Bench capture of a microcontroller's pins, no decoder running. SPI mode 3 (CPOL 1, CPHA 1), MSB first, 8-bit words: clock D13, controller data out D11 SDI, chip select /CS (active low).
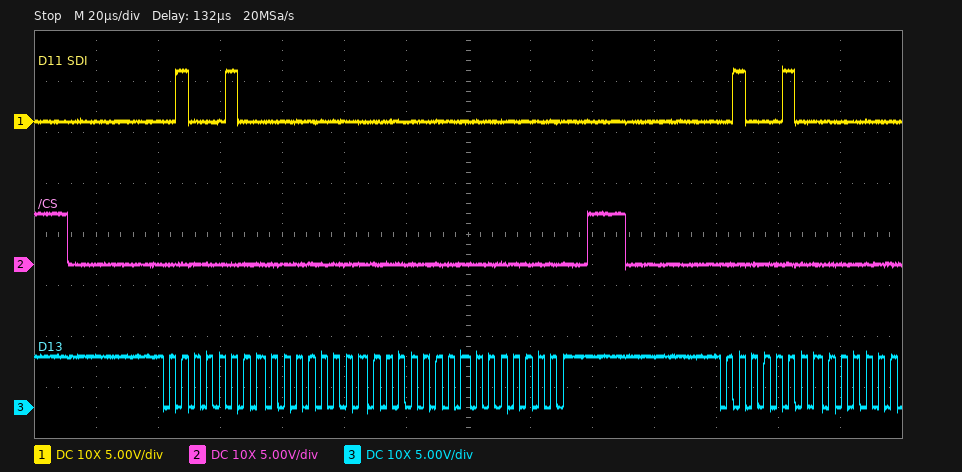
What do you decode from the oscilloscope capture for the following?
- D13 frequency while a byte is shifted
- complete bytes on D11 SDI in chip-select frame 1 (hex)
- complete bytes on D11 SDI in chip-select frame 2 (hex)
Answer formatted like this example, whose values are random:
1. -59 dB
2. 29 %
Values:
1. 250 kHz
2. 44 00 00 00
3. 44
